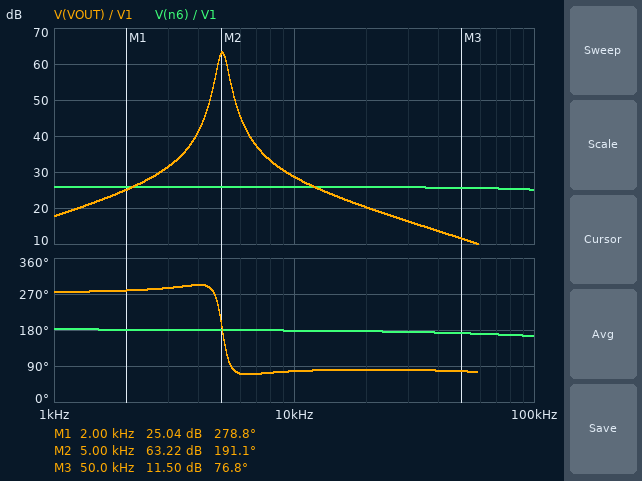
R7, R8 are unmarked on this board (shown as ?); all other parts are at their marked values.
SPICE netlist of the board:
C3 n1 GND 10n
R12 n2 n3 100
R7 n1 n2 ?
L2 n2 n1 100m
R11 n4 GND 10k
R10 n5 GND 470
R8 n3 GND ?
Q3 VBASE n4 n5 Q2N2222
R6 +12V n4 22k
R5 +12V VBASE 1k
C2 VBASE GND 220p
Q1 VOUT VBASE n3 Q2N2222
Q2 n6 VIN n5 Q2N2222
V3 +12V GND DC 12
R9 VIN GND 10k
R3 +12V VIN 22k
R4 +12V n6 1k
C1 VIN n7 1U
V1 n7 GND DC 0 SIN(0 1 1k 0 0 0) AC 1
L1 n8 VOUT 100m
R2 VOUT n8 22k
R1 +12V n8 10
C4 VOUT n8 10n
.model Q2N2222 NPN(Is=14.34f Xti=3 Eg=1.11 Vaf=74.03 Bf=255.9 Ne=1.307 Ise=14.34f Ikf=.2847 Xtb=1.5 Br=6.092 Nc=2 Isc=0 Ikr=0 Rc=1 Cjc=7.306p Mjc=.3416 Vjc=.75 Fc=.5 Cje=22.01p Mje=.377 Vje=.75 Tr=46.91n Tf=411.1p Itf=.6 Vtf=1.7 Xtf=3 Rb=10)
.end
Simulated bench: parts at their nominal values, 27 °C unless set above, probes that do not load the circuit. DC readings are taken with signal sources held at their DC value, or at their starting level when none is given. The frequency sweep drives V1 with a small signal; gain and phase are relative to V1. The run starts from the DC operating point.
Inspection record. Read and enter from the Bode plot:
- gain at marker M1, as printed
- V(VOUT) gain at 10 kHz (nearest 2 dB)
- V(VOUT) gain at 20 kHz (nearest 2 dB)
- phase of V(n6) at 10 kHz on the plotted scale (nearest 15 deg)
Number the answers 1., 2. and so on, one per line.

1. 25.04 dB
2. 28 dB
3. 20 dB
4. 180 deg
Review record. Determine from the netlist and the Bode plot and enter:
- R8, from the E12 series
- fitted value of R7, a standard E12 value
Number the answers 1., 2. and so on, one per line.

1. 1.5 kΩ
2. 56 kΩ
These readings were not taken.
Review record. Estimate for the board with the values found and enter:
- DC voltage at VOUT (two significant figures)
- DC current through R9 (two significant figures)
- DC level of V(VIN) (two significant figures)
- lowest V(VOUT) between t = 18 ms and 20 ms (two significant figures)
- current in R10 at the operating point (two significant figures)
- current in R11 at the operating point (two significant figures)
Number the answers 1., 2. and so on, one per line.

1. 12 V
2. 360 µA
3. 3.6 V
4. 3.1 V
5. 6.3 mA
6. 360 µA
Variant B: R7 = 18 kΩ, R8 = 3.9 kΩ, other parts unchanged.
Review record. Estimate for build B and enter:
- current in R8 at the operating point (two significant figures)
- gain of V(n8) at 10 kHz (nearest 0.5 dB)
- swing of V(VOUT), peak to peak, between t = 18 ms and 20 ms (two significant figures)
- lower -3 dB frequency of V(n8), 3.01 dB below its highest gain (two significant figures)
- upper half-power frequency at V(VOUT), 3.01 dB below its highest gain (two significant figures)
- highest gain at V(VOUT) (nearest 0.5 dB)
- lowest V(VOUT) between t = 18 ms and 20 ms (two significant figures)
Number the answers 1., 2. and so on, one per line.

1. 2.1 mA
2. -23.0 dB
3. 16 V
4. 4.5 kHz
5. 5.3 kHz
6. 56.5 dB
7. 4.2 V
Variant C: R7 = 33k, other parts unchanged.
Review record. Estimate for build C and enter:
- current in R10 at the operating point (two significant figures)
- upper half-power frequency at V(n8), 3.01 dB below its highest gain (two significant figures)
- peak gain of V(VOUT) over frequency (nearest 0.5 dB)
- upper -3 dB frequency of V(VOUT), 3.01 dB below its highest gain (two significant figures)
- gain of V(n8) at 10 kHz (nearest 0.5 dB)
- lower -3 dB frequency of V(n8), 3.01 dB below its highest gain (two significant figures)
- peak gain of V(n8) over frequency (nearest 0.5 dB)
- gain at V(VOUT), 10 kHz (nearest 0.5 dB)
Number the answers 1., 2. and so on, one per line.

1. 6.3 mA
2. 5.4 kHz
3. 61.0 dB
4. 5.3 kHz
5. -17.5 dB
6. 4.7 kHz
7. -6.0 dB
8. 29.0 dB
